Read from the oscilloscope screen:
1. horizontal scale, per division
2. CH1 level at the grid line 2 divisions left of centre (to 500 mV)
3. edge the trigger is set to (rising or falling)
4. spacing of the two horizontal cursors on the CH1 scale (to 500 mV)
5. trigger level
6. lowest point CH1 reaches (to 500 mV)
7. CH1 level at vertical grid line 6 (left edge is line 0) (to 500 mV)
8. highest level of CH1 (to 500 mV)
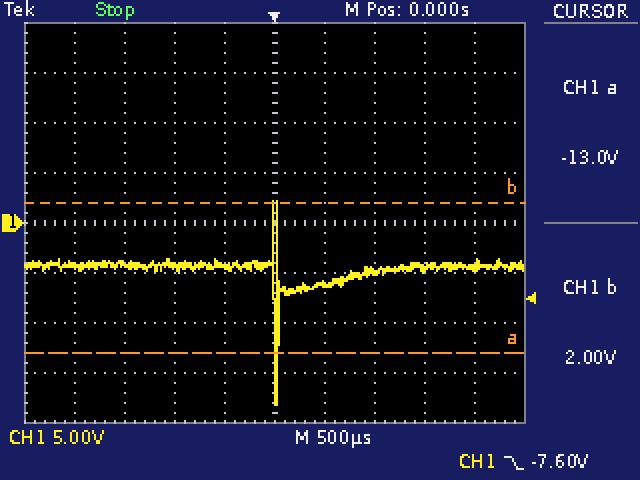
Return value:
500 µs
-4.5 V
falling
15.0 V
-7.60 V
-18.0 V
-6.0 V
2.0 V
